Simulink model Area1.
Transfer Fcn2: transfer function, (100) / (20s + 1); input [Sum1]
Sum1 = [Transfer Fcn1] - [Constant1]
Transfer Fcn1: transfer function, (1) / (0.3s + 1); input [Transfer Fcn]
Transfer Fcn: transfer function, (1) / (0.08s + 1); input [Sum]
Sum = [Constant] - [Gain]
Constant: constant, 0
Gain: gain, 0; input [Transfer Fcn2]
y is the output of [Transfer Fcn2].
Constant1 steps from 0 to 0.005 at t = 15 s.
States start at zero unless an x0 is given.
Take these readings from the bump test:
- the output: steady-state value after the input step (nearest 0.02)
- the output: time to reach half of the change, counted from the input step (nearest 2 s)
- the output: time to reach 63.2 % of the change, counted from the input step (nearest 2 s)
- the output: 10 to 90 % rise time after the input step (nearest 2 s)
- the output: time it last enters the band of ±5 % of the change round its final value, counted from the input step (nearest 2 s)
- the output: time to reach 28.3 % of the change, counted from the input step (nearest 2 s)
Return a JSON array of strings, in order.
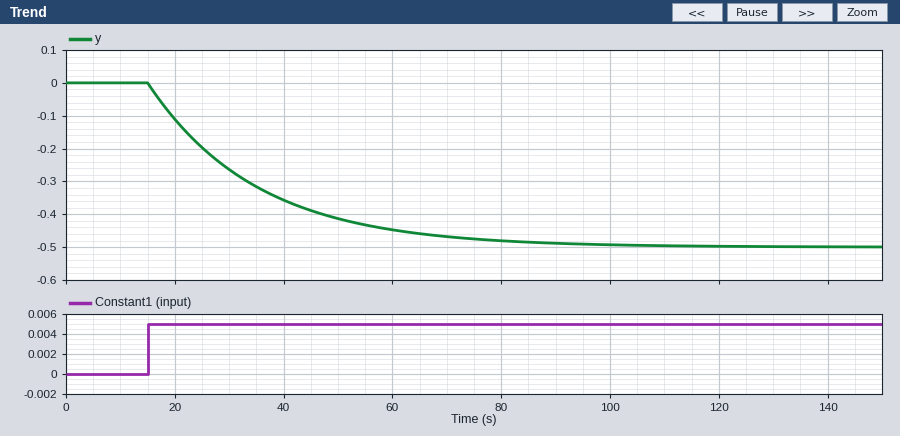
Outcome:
["-0.50", "14 s", "20 s", "44 s", "60 s", "6 s"]
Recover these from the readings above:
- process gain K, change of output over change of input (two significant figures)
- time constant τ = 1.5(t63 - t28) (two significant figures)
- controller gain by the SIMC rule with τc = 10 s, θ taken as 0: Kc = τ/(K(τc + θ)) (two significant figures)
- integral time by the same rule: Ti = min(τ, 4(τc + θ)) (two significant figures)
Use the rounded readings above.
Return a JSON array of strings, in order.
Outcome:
["-100", "21 s", "-0.021", "21 s"]
